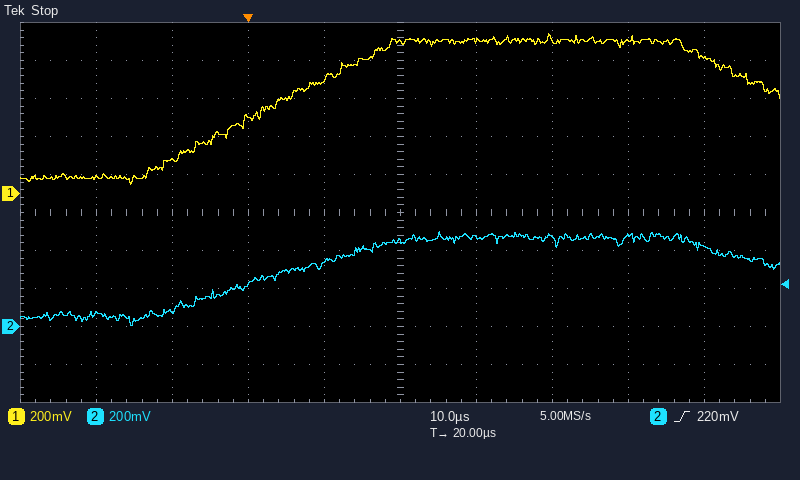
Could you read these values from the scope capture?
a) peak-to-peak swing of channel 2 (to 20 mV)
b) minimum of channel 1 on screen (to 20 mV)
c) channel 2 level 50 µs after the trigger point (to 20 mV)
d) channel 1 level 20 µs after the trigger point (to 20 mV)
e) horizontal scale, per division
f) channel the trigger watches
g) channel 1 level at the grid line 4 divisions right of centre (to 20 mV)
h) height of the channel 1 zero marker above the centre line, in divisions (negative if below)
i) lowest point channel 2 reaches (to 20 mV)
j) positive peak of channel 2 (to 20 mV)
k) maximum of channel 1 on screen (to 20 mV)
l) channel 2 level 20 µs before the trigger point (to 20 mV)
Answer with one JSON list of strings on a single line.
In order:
["500 mV", "40 mV", "480 mV", "800 mV", "10 µs", "channel 2", "720 mV", "+0.5 div", "0 mV", "500 mV", "840 mV", "60 mV"]
